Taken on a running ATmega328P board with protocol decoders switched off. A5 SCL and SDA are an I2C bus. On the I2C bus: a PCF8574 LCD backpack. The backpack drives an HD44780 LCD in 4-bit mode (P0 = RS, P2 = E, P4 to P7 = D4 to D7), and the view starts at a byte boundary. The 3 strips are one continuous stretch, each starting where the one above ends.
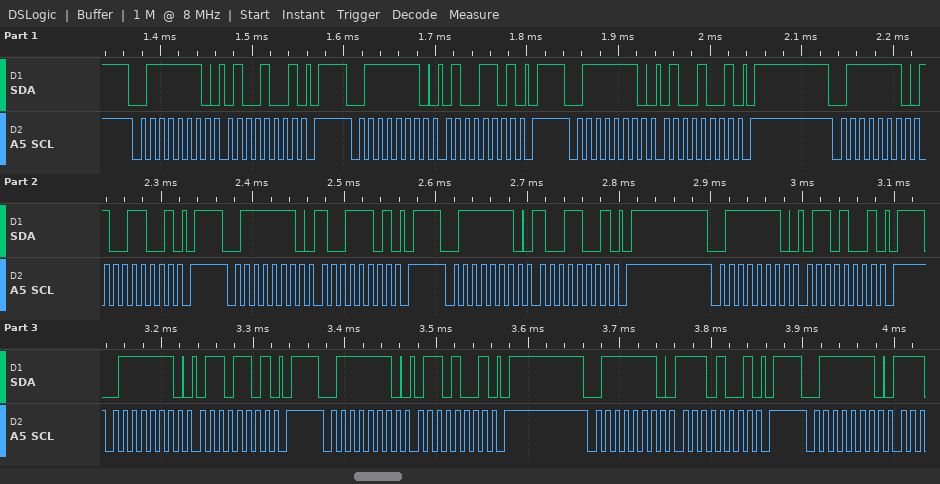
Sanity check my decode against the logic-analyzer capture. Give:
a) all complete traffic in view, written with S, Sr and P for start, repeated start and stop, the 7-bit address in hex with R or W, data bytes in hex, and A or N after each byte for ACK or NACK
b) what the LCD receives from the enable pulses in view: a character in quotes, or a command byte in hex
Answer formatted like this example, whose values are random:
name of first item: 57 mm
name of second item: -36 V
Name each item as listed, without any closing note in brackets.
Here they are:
all complete traffic in view, written with S, Sr and P for start, repeated start and stop, the 7-bit address in hex with R or W, data bytes in hex, and A or N after each byte for ACK or NACK: S 3FW A 49 A P S 3FW A 4D A P S 3FW A 49 A P S 3FW A 99 A P S 3FW A 9D A P S 3FW A 99 A P S 3FW A 69 A P S 3FW A 6D A P S 3FW A 69 A P S 3FW A E9 A P S 3FW A
what the LCD receives from the enable pulses in view: a character in quotes, or a command byte in hex: 'I'
